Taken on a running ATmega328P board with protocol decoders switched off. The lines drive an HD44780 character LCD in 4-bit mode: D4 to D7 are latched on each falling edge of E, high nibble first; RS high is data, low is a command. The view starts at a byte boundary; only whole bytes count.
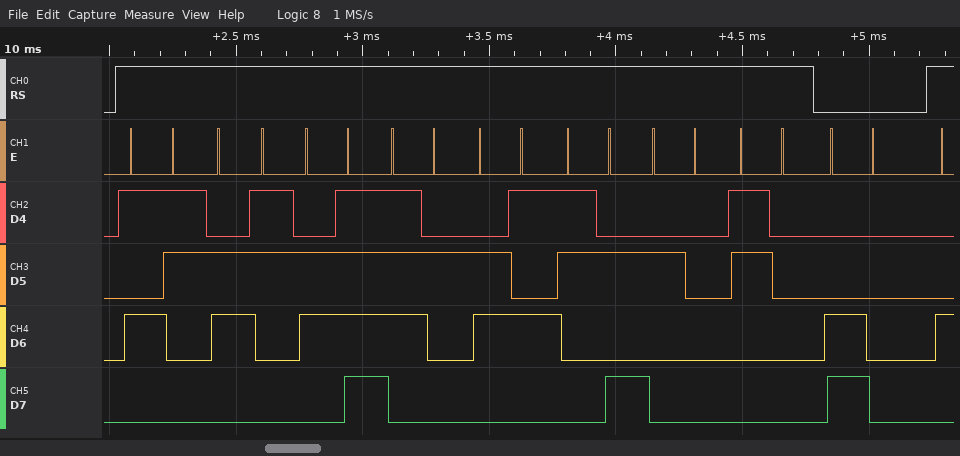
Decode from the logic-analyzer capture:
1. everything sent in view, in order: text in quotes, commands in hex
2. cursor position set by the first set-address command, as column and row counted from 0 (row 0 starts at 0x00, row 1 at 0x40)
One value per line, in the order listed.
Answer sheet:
"Score: 0" 0xC0
column 0, row 1
